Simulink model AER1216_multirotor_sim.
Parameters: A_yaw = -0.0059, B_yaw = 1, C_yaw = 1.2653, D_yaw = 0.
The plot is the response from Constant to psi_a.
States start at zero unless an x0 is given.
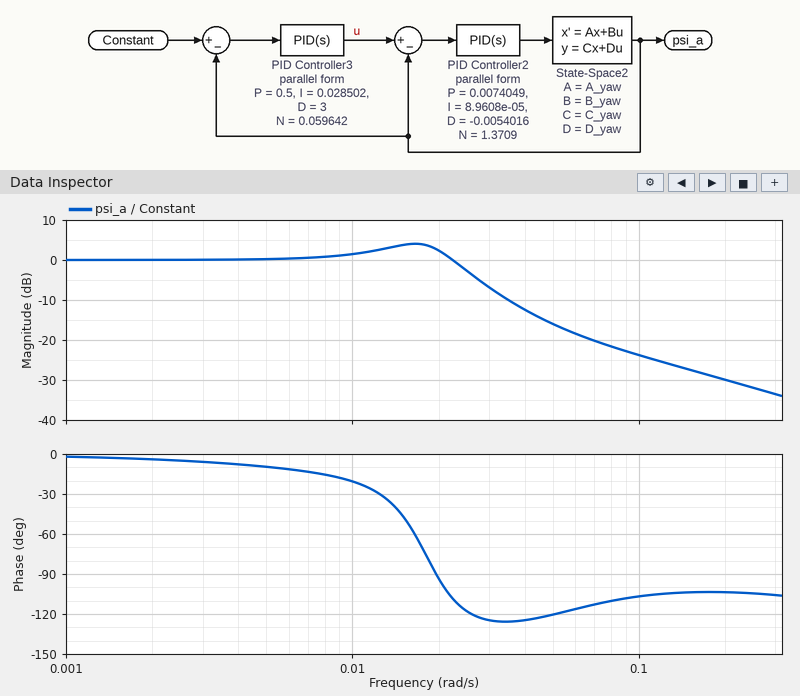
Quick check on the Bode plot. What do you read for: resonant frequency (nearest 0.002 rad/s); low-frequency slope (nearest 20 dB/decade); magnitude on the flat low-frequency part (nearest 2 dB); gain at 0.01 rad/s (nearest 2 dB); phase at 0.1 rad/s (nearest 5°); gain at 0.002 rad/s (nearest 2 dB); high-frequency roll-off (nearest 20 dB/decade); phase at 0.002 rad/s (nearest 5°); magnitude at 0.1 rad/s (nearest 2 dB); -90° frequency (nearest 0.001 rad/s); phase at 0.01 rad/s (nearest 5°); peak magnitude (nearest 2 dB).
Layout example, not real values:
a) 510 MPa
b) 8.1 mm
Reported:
a) 0.016 rad/s
b) 0 dB/decade
c) 0 dB
d) 2 dB
e) -105°
f) 0 dB
g) -20 dB/decade
h) -5°
i) -24 dB
j) 0.020 rad/s
k) -20°
l) 4 dB
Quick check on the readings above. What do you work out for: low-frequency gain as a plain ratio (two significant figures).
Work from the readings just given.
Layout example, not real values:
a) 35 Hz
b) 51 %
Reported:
a) 1.0
